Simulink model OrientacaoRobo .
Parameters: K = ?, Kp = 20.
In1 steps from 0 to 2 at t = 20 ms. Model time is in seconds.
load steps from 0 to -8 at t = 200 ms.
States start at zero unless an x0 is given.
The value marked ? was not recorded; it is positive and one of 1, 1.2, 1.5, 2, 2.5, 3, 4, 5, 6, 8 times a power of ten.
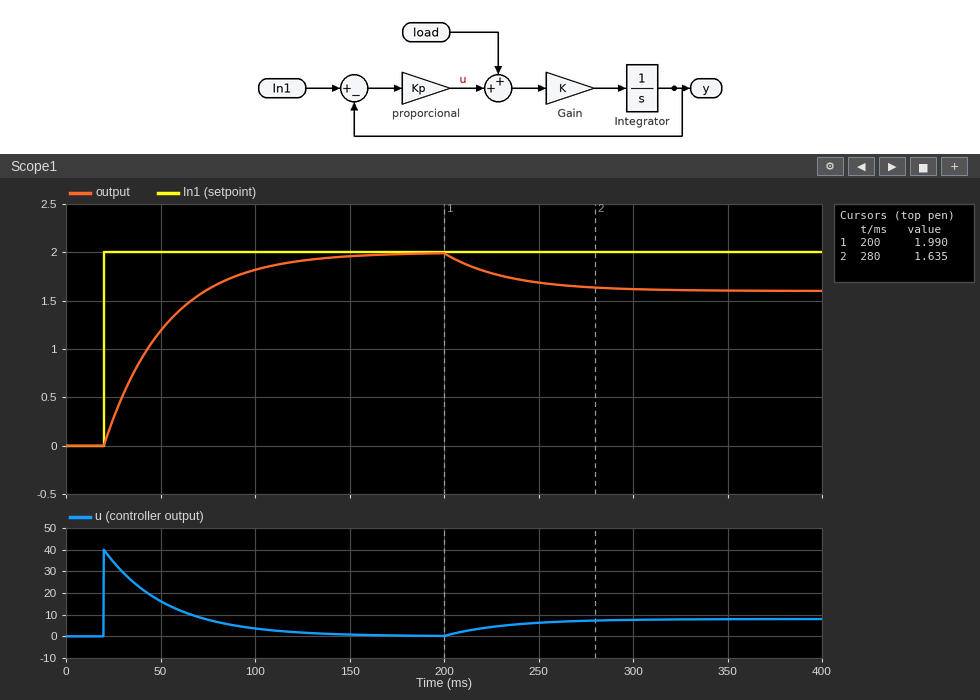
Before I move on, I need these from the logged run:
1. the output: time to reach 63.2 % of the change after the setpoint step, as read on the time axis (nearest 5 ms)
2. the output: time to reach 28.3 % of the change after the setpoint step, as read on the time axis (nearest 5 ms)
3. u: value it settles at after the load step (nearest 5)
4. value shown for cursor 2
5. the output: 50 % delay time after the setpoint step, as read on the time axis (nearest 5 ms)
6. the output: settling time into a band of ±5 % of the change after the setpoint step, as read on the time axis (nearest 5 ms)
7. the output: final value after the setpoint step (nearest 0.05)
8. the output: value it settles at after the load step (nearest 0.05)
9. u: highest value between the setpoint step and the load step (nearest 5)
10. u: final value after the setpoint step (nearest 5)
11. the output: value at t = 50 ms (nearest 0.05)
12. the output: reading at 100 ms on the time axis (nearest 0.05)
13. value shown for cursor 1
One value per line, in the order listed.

55 ms
30 ms
10
1.635
45 ms
120 ms
2.00
1.60
40
0
1.20
1.80
1.990
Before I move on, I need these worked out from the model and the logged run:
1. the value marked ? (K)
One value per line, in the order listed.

1.5
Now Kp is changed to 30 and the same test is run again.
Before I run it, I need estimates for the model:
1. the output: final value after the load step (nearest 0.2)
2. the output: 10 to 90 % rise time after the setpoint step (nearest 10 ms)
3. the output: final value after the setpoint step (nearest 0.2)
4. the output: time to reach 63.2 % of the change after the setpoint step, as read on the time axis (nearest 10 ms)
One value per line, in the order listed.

1.8
50 ms
2.0
40 ms
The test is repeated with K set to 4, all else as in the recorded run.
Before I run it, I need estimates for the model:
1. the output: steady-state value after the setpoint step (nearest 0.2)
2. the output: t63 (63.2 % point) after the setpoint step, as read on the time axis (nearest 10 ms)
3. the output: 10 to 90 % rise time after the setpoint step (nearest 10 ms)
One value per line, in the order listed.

2.0
30 ms
30 ms
